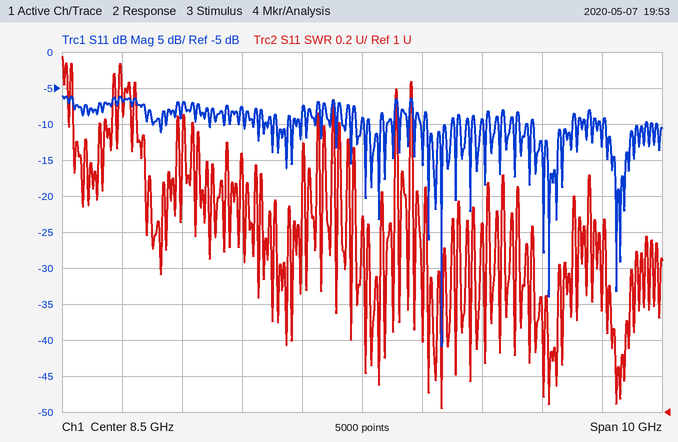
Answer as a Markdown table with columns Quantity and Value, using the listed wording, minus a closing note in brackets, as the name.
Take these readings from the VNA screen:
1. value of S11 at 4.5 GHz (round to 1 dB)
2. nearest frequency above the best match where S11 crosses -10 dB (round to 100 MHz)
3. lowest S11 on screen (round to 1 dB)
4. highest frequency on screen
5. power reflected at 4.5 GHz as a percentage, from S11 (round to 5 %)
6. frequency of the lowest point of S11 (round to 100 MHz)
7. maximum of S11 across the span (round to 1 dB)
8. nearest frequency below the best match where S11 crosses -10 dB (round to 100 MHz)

| Quantity | Value |
|---|---|
| value of S11 at 4.5 GHz | -7 dB |
| nearest frequency above the best match where S11 crosses -10 dB | 10.0 GHz |
| lowest S11 on screen | -41 dB |
| highest frequency on screen | 13.5 GHz |
| power reflected at 4.5 GHz as a percentage, from S11 | 20 % |
| frequency of the lowest point of S11 | 9.8 GHz |
| maximum of S11 across the span | -6 dB |
| nearest frequency below the best match where S11 crosses -10 dB | 9.6 GHz |
